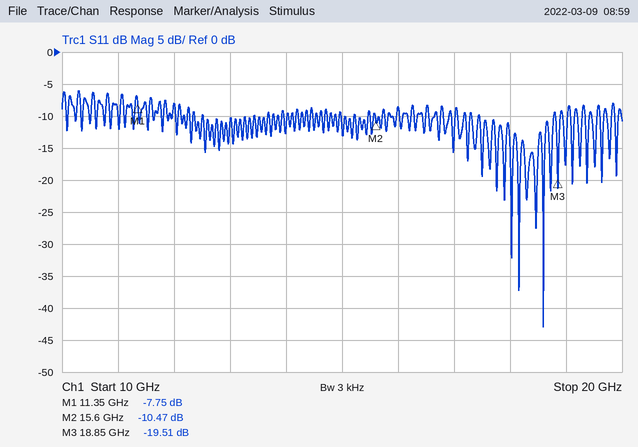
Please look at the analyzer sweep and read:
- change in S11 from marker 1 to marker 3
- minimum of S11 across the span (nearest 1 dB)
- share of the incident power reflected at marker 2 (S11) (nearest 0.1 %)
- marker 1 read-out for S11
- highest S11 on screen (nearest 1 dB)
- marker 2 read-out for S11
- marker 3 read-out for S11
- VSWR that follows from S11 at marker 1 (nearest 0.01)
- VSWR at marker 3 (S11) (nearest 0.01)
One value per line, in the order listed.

-11.76 dB
-43 dB
9.0 %
-7.75 dB
-6 dB
-10.47 dB
-19.51 dB
2.39
1.24
